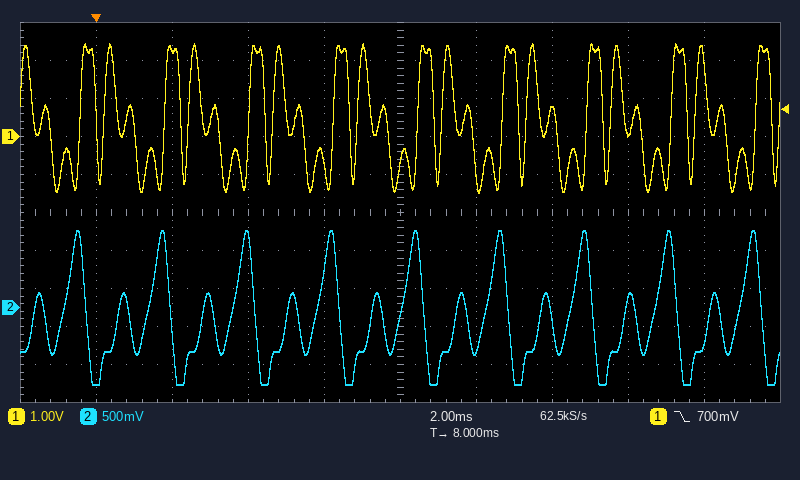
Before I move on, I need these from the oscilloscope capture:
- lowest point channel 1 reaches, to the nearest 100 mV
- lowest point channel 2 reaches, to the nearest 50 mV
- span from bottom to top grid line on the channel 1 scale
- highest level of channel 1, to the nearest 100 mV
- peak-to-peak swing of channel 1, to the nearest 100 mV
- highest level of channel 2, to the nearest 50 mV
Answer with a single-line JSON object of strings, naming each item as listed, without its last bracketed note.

{"lowest point channel 1 reaches, to the nearest 100 mV": "-1.5 V", "lowest point channel 2 reaches, to the nearest 50 mV": "-1.00 V", "span from bottom to top grid line on the channel 1 scale": "10 V", "highest level of channel 1, to the nearest 100 mV": "2.4 V", "peak-to-peak swing of channel 1, to the nearest 100 mV": "3.9 V", "highest level of channel 2, to the nearest 50 mV": "1.00 V"}
